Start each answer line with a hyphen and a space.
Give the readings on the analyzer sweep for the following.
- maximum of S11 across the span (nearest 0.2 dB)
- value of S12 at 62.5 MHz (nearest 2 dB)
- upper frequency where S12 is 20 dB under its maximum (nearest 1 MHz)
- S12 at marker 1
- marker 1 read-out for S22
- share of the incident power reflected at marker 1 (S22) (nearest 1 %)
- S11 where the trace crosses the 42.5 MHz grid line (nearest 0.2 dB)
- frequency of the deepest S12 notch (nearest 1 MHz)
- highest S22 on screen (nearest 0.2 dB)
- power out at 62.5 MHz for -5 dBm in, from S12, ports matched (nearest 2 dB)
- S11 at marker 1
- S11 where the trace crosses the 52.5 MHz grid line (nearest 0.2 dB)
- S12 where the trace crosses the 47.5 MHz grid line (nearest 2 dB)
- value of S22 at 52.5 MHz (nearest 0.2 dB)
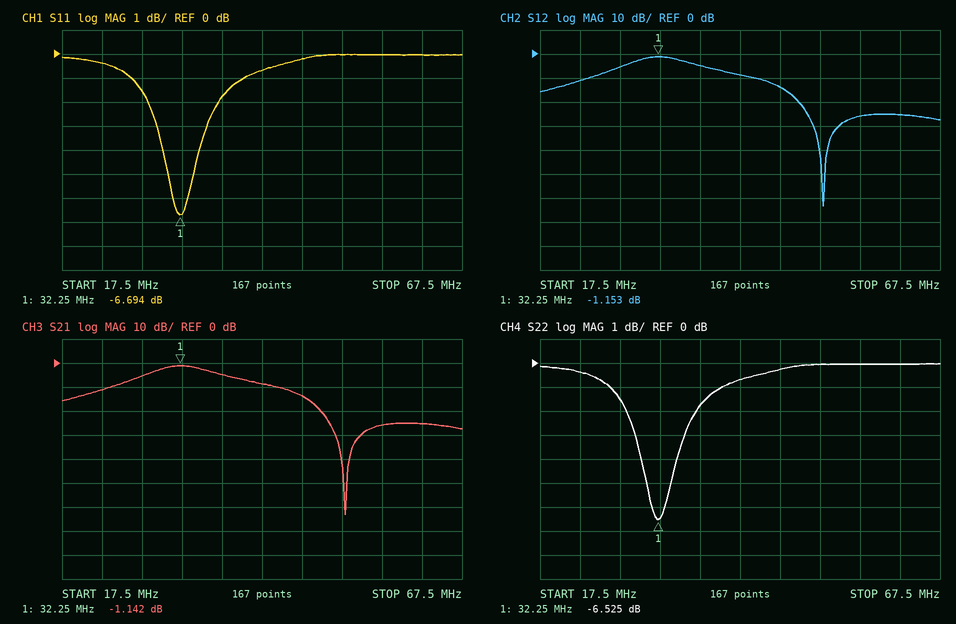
- 0.0 dB
- -26 dB
- 50 MHz
- -1.153 dB
- -6.525 dB
- 22 %
- -0.6 dB
- 53 MHz
- 0.0 dB
- -30 dBm
- -6.694 dB
- 0.0 dB
- -14 dB
- 0.0 dB
